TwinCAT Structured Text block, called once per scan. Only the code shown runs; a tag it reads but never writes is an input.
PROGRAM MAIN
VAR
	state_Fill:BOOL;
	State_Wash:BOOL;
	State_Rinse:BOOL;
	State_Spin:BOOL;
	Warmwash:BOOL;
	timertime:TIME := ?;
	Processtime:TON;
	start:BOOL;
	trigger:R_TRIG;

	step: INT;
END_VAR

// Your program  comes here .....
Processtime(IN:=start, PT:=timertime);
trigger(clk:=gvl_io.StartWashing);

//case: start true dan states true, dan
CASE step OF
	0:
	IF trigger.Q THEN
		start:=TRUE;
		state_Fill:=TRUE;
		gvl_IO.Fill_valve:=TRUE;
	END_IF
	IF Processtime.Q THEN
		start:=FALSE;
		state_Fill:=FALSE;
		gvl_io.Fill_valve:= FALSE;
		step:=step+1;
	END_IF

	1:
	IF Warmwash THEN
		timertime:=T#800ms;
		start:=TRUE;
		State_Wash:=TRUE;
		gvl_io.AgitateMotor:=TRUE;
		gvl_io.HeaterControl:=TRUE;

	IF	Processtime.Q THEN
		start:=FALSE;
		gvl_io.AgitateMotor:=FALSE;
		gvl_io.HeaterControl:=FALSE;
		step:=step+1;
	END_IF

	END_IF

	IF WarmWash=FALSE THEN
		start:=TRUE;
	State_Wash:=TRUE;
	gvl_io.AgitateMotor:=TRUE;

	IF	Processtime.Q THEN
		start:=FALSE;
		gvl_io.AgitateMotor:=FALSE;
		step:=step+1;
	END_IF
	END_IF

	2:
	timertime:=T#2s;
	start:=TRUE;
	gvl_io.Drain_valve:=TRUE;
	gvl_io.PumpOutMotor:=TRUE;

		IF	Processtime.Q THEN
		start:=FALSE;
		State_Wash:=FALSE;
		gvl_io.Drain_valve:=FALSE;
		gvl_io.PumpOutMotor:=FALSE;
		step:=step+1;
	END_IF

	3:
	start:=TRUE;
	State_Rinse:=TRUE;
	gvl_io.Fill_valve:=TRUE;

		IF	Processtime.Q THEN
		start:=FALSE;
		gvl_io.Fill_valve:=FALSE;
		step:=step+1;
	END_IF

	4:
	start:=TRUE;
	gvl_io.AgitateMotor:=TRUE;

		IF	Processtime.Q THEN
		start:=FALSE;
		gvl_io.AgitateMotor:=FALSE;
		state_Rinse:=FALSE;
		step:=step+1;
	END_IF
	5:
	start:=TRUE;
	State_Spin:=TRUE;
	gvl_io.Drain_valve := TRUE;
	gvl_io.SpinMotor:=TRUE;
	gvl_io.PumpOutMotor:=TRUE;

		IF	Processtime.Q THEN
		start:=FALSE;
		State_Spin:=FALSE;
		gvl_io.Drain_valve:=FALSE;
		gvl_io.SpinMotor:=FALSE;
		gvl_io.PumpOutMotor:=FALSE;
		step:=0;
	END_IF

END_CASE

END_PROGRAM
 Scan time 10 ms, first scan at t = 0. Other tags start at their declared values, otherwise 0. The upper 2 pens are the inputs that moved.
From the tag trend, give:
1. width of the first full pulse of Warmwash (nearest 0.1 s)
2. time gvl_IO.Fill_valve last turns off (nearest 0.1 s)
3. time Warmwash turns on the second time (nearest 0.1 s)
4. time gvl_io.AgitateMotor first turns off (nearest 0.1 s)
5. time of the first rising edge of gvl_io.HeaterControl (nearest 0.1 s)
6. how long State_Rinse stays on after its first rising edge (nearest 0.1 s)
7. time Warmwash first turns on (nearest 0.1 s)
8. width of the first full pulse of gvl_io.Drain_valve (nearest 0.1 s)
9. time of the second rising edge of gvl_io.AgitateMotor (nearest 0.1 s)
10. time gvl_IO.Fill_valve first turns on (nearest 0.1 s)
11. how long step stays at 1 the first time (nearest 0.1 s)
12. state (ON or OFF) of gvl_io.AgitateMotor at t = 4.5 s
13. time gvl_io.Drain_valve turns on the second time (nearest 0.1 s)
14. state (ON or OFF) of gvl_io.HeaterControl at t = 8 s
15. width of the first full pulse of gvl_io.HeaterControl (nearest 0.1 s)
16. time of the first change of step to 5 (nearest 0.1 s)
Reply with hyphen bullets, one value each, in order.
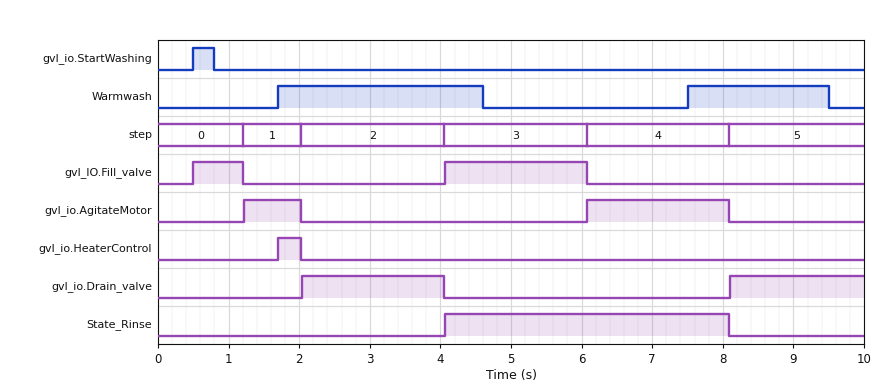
- 2.9 s
- 6.1 s
- 7.5 s
- 2.0 s
- 1.7 s
- 4.0 s
- 1.7 s
- 2.0 s
- 6.1 s
- 0.5 s
- 0.8 s
- OFF
- 8.1 s
- OFF
- 0.3 s
- 8.1 s
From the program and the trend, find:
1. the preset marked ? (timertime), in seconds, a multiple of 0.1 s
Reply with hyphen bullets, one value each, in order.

- 0.7 s
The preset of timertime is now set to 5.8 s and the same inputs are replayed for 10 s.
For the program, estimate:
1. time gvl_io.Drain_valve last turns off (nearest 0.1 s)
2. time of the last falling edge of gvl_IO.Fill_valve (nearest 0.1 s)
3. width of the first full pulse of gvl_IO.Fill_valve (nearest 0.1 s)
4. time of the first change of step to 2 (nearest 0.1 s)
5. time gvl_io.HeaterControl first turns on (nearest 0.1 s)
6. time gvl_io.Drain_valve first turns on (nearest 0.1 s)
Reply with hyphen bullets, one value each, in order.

- 9.5 s
- 6.3 s
- 5.8 s
- 7.5 s
- 7.5 s
- 7.5 s
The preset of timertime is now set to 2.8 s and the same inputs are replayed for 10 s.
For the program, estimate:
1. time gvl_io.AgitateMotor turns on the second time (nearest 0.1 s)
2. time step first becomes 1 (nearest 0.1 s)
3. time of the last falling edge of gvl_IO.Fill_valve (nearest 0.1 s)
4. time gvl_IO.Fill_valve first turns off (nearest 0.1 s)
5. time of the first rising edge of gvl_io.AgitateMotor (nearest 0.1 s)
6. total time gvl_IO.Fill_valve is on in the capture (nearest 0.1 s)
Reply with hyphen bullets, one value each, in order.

- 8.2 s
- 3.3 s
- 8.2 s
- 3.3 s
- 3.3 s
- 4.8 s
